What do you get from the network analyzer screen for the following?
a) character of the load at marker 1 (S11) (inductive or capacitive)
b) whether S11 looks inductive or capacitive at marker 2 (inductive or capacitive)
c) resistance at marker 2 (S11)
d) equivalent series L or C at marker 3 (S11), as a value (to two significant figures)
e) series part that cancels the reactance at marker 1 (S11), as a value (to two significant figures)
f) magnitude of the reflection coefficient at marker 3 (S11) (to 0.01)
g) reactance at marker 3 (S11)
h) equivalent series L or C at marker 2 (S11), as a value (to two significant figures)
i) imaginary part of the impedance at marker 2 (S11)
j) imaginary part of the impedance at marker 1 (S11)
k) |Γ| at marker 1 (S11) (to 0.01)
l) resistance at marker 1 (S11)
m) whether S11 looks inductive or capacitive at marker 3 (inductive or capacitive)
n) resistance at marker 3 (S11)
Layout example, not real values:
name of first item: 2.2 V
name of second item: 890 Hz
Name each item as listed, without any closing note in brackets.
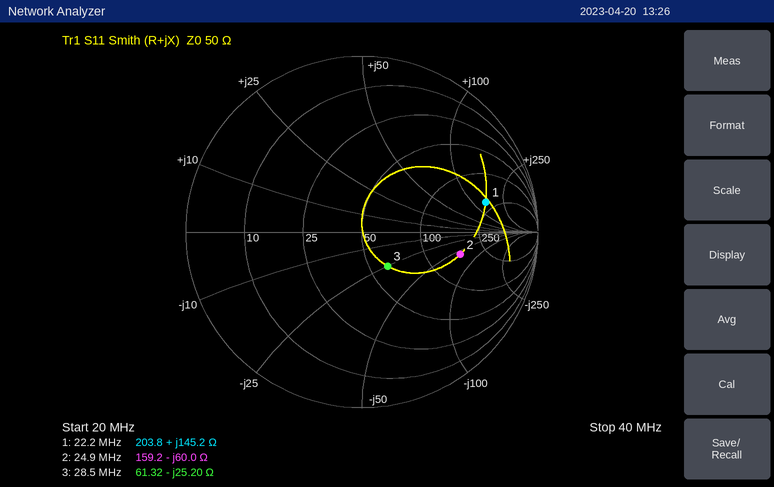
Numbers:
character of the load at marker 1 (S11): inductive
whether S11 looks inductive or capacitive at marker 2: capacitive
resistance at marker 2: 159.2 Ω
equivalent series L or C at marker 3 (S11), as a value: 220 pF
series part that cancels the reactance at marker 1 (S11), as a value: 49 pF
magnitude of the reflection coefficient at marker 3 (S11): 0.24
reactance at marker 3: -25.20 Ω
equivalent series L or C at marker 2 (S11), as a value: 110 pF
imaginary part of the impedance at marker 2: -60.0 Ω
imaginary part of the impedance at marker 1: +145.2 Ω
|Γ| at marker 1 (S11): 0.72
resistance at marker 1: 203.8 Ω
whether S11 looks inductive or capacitive at marker 3: capacitive
resistance at marker 3: 61.32 Ω
